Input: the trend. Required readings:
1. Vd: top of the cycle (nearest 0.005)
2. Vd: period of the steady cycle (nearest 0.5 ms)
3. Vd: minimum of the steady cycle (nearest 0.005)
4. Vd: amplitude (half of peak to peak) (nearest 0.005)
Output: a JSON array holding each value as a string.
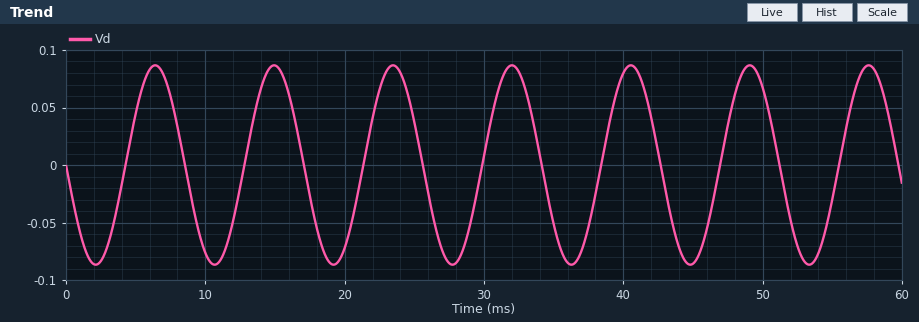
["0.085", "8.5 ms", "-0.085", "0.085"]
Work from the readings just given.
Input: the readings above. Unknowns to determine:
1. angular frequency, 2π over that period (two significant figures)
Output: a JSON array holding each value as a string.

["0.74 rad/ms"]
